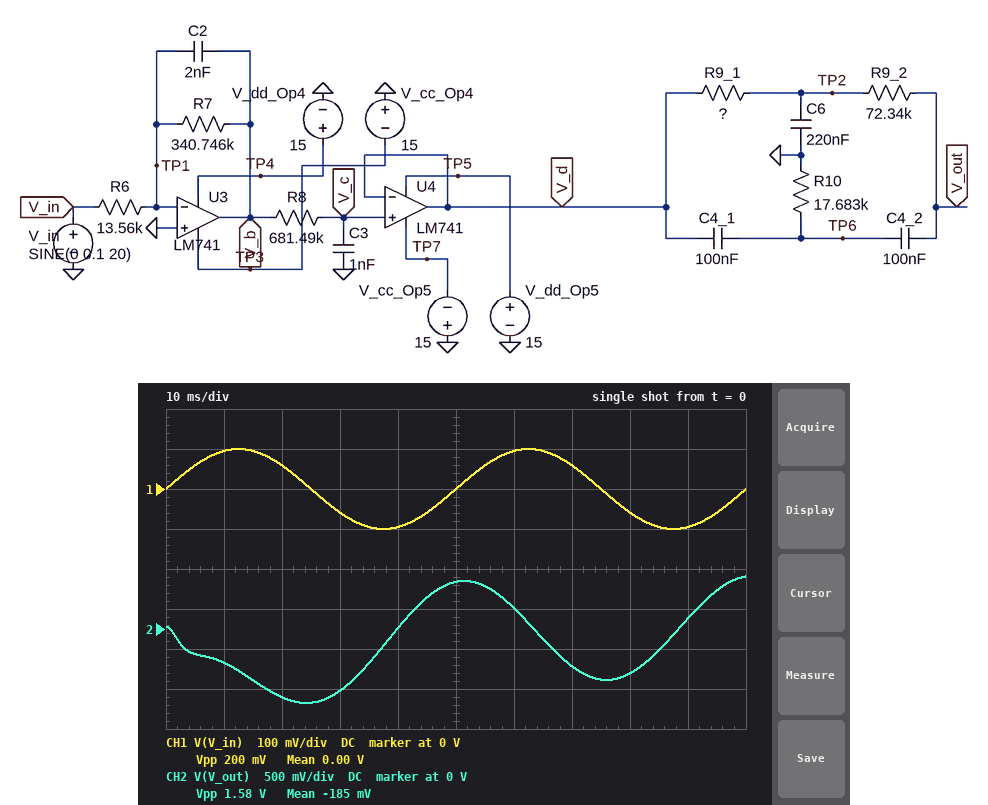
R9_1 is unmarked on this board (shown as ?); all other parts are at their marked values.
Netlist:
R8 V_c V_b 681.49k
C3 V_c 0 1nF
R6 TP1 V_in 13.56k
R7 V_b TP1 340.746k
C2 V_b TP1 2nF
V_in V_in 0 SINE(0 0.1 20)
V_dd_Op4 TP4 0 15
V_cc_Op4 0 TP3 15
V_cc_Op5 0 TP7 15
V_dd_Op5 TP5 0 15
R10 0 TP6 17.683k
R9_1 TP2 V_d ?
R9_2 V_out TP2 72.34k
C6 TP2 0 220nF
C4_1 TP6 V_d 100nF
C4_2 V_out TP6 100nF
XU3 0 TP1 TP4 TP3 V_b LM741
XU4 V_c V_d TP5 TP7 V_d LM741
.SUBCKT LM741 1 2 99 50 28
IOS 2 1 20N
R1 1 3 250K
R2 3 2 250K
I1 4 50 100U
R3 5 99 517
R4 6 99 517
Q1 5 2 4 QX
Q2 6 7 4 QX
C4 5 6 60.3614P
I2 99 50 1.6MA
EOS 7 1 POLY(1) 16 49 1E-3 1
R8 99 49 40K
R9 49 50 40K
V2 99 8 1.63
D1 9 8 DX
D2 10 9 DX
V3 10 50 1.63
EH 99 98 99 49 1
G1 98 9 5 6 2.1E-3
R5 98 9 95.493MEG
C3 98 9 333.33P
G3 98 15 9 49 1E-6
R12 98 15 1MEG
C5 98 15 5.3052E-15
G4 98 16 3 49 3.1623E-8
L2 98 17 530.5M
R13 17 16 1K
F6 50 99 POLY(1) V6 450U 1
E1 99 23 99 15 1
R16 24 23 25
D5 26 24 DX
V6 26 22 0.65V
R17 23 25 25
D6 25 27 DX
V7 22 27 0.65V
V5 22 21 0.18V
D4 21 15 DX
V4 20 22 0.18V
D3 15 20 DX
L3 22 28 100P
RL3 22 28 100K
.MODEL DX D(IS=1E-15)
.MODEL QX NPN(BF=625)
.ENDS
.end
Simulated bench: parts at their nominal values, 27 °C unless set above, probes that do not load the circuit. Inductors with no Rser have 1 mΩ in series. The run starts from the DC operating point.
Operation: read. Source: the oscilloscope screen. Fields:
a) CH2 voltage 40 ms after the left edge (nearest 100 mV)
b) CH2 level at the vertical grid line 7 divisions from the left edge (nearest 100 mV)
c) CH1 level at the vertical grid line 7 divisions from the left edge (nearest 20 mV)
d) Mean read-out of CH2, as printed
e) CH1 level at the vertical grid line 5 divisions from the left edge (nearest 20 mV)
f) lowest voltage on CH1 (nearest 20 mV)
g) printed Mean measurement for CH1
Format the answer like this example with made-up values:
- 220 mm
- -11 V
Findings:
- 0 V
- -500 mV
- 60 mV
- -185 mV
- 0 V
- -100 mV
- 0.00 V
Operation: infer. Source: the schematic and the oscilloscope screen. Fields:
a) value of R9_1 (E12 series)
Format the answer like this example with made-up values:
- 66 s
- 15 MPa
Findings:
- 39 kΩ
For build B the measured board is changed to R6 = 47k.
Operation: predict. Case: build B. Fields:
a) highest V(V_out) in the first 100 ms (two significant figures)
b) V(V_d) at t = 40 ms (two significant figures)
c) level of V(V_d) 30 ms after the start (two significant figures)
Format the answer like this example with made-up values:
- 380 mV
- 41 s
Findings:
- 190 mV
- 720 mV
- 320 mV
